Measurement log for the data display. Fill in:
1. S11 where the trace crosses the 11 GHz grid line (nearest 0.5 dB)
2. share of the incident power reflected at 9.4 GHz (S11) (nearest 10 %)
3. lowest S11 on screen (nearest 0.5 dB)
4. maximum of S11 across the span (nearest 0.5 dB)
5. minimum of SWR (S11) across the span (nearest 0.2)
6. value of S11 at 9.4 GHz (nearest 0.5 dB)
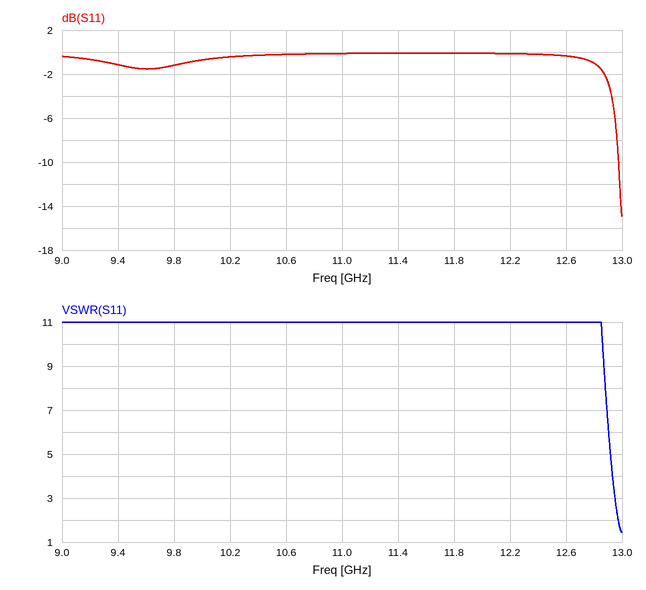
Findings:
0.0 dB
80 %
-15.0 dB
0.0 dB
1.4
-1.0 dB
